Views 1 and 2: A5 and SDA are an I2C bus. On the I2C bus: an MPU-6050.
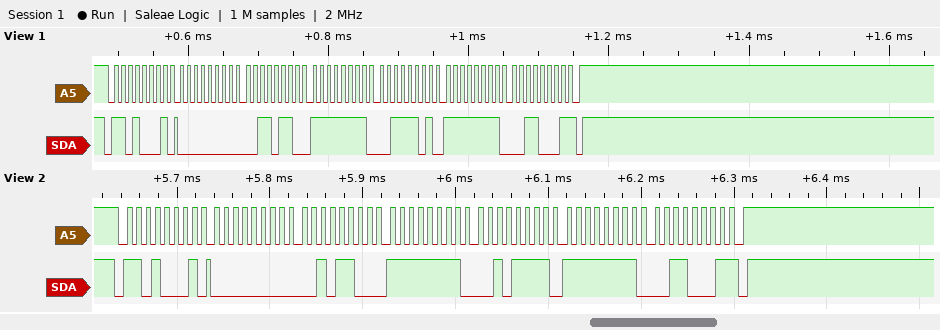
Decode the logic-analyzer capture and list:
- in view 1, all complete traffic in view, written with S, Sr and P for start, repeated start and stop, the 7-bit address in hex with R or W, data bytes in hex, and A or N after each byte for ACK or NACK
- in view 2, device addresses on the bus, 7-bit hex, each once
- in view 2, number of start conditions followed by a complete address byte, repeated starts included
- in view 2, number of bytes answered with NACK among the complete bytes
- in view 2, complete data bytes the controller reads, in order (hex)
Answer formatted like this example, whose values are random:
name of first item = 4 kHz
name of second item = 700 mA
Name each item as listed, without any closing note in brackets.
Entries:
in view 1, all complete traffic in view, written with S, Sr and P for start, repeated start and stop, the 7-bit address in hex with R or W, data bytes in hex, and A or N after each byte for ACK or NACK = S 68R A 00 A 36 A FF A 3D A FF A 31 N P
in view 2, device addresses on the bus, 7-bit hex, each once = 0x68
in view 2, number of start conditions followed by a complete address byte, repeated starts included = 1
in view 2, number of bytes answered with NACK among the complete bytes = 1
in view 2, complete data bytes the controller reads, in order = 00 2C FF 2F FF 31
